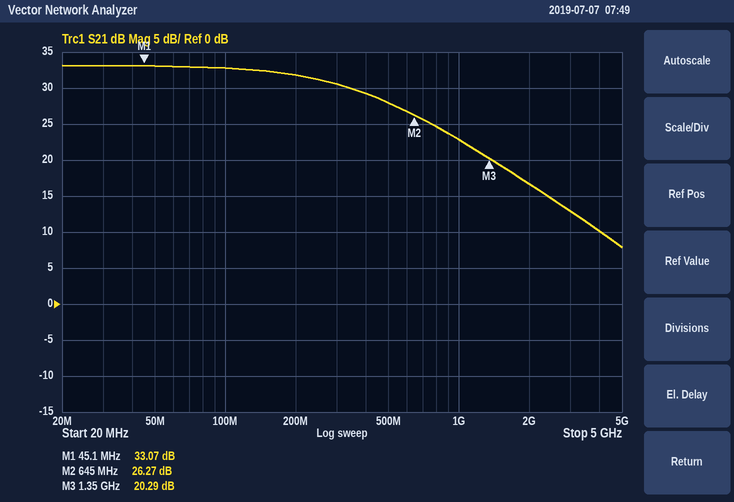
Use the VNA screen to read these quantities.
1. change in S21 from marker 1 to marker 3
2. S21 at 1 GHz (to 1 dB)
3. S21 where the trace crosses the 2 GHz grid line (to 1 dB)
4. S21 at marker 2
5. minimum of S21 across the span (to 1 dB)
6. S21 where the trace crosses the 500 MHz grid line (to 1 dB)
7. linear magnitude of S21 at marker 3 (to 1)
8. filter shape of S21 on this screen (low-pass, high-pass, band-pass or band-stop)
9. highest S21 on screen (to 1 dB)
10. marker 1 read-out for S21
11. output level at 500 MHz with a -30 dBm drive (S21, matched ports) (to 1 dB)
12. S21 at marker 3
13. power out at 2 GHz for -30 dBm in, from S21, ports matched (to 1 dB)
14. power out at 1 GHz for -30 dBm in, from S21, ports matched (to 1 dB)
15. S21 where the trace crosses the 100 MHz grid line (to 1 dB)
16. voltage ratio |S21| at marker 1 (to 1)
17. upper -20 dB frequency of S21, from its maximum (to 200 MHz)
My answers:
-12.78 dB
23 dB
17 dB
26.27 dB
8 dB
28 dB
10
low-pass
33 dB
33.07 dB
-2 dBm
20.29 dB
-13 dBm
-7 dBm
33 dB
45
3.0 GHz
